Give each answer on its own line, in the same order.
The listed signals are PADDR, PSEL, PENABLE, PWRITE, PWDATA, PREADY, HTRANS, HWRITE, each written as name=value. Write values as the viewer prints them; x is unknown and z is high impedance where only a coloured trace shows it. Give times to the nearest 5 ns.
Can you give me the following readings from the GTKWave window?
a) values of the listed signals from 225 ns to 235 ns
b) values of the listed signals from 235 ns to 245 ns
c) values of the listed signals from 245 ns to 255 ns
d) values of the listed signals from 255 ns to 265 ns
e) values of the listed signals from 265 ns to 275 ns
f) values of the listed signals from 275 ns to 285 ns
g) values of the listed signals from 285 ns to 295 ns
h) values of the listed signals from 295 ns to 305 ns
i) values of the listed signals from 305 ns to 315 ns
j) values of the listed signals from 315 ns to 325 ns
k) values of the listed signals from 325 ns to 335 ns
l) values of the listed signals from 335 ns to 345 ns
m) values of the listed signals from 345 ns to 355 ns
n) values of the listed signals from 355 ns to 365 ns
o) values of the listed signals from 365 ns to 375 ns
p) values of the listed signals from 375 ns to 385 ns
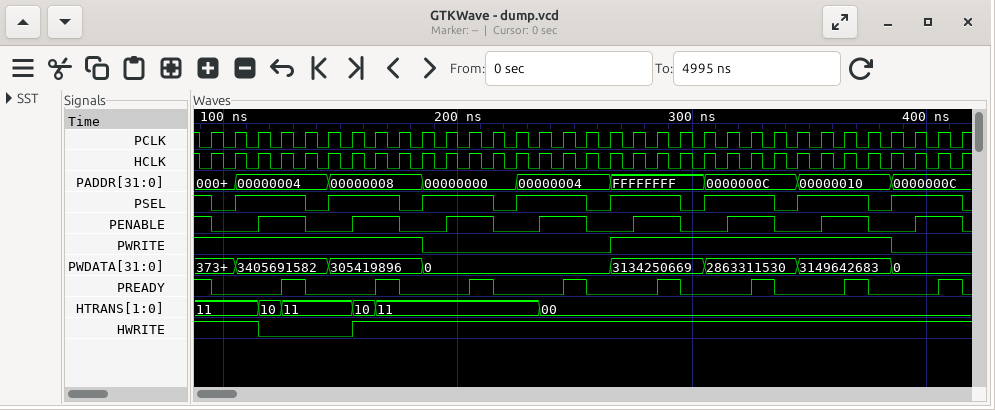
PADDR=00000004, PSEL=1, PENABLE=0, PWRITE=0, PWDATA=0, PREADY=0, HTRANS=11, HWRITE=1
PADDR=00000004, PSEL=1, PENABLE=1, PWRITE=0, PWDATA=0, PREADY=0, HTRANS=00, HWRITE=1
PADDR=00000004, PSEL=1, PENABLE=1, PWRITE=0, PWDATA=0, PREADY=1, HTRANS=00, HWRITE=1
PADDR=00000004, PSEL=0, PENABLE=0, PWRITE=0, PWDATA=0, PREADY=0, HTRANS=00, HWRITE=1
PADDR=FFFFFFFF, PSEL=1, PENABLE=0, PWRITE=1, PWDATA=3134250669, PREADY=0, HTRANS=00, HWRITE=1
PADDR=FFFFFFFF, PSEL=1, PENABLE=1, PWRITE=1, PWDATA=3134250669, PREADY=0, HTRANS=00, HWRITE=1
PADDR=FFFFFFFF, PSEL=1, PENABLE=1, PWRITE=1, PWDATA=3134250669, PREADY=1, HTRANS=00, HWRITE=1
PADDR=FFFFFFFF, PSEL=0, PENABLE=0, PWRITE=1, PWDATA=3134250669, PREADY=0, HTRANS=00, HWRITE=1
PADDR=0000000C, PSEL=1, PENABLE=0, PWRITE=1, PWDATA=2863311530, PREADY=0, HTRANS=00, HWRITE=1
PADDR=0000000C, PSEL=1, PENABLE=1, PWRITE=1, PWDATA=2863311530, PREADY=0, HTRANS=00, HWRITE=1
PADDR=0000000C, PSEL=1, PENABLE=1, PWRITE=1, PWDATA=2863311530, PREADY=1, HTRANS=00, HWRITE=1
PADDR=0000000C, PSEL=0, PENABLE=0, PWRITE=1, PWDATA=2863311530, PREADY=0, HTRANS=00, HWRITE=1
PADDR=00000010, PSEL=1, PENABLE=0, PWRITE=1, PWDATA=3149642683, PREADY=0, HTRANS=00, HWRITE=1
PADDR=00000010, PSEL=1, PENABLE=1, PWRITE=1, PWDATA=3149642683, PREADY=0, HTRANS=00, HWRITE=1
PADDR=00000010, PSEL=1, PENABLE=1, PWRITE=1, PWDATA=3149642683, PREADY=1, HTRANS=00, HWRITE=1
PADDR=00000010, PSEL=0, PENABLE=0, PWRITE=1, PWDATA=3149642683, PREADY=0, HTRANS=00, HWRITE=1
